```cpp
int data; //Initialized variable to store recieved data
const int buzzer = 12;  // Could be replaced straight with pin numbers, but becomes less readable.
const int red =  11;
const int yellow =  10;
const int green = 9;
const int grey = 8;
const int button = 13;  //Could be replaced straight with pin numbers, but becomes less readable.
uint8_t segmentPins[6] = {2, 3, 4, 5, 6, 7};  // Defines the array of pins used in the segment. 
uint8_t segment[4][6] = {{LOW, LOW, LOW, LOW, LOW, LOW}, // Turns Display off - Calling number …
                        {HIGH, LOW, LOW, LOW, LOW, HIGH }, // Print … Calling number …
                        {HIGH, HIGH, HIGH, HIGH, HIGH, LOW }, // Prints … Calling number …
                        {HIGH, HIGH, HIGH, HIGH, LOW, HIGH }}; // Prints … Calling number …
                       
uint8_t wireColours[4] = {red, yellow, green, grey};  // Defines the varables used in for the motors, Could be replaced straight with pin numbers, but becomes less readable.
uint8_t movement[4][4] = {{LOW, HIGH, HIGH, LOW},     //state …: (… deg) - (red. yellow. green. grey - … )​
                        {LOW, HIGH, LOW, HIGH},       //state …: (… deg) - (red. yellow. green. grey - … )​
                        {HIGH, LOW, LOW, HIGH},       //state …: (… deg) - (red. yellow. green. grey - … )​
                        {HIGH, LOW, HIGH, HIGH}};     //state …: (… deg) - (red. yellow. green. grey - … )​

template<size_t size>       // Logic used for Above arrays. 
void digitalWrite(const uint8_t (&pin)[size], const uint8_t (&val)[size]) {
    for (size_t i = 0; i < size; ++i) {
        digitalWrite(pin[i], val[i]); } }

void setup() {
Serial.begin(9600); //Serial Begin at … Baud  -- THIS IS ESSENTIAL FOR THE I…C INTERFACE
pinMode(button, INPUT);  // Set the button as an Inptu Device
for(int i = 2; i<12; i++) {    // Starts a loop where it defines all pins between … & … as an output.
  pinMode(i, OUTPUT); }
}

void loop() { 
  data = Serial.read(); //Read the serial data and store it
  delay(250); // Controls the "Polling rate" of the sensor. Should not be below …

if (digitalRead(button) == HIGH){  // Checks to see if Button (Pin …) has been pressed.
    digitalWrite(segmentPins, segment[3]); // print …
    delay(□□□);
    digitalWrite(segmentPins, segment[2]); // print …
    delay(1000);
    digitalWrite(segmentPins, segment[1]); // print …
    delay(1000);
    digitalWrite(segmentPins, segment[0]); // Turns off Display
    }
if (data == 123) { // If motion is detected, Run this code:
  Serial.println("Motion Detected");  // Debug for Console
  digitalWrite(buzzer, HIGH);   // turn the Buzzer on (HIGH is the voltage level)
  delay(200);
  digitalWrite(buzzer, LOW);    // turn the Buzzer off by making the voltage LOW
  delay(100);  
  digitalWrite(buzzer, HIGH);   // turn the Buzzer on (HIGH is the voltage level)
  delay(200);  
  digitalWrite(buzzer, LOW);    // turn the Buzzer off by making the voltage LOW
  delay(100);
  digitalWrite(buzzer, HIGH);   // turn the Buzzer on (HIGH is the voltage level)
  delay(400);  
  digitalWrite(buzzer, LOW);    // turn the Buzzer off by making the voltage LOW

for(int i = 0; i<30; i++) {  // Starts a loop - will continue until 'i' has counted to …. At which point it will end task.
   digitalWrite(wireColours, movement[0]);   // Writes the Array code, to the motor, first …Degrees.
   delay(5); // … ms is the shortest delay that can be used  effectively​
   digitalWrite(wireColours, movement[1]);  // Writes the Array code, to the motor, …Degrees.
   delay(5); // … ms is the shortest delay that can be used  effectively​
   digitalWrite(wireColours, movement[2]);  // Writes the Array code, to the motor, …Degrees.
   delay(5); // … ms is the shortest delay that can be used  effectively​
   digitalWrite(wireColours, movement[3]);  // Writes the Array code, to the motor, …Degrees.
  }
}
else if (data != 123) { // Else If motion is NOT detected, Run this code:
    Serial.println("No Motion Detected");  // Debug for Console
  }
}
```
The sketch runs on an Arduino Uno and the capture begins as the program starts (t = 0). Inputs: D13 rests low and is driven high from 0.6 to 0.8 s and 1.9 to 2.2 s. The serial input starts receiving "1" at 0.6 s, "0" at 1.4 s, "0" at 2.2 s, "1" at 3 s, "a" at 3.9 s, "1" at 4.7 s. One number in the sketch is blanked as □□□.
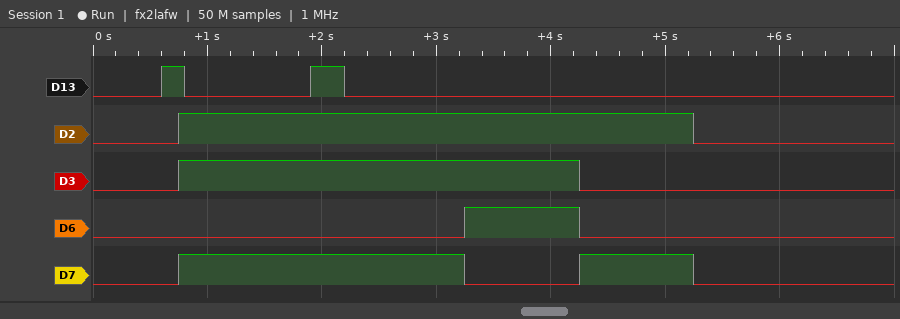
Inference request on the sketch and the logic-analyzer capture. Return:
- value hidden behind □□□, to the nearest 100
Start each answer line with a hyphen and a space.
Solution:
- 2500
